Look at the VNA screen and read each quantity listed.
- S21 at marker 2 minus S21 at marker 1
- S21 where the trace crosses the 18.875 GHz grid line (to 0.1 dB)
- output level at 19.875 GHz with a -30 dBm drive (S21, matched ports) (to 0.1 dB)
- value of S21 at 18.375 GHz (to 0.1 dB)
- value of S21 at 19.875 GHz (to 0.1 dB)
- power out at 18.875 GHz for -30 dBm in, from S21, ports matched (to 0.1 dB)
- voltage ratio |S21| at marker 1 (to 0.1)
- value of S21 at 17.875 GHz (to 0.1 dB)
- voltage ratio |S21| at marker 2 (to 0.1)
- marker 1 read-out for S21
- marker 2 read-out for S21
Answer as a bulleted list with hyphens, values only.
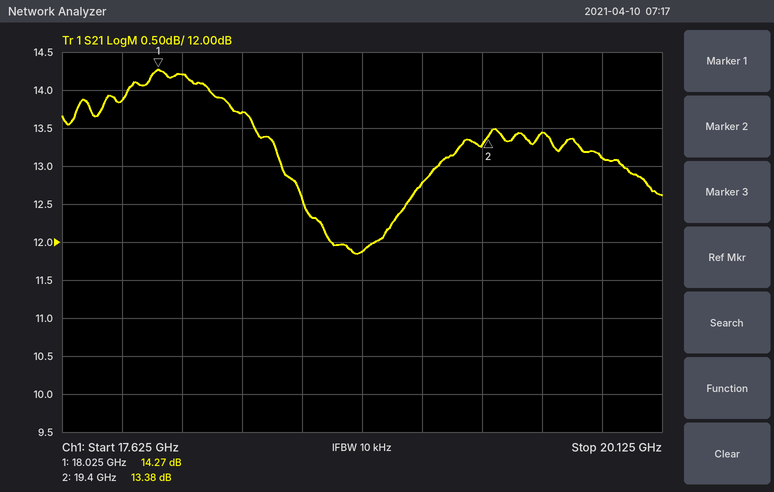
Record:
- -0.89 dB
- 11.9 dB
- -16.9 dBm
- 13.7 dB
- 13.1 dB
- -18.1 dBm
- 5.2
- 13.9 dB
- 4.7
- 14.27 dB
- 13.38 dB
